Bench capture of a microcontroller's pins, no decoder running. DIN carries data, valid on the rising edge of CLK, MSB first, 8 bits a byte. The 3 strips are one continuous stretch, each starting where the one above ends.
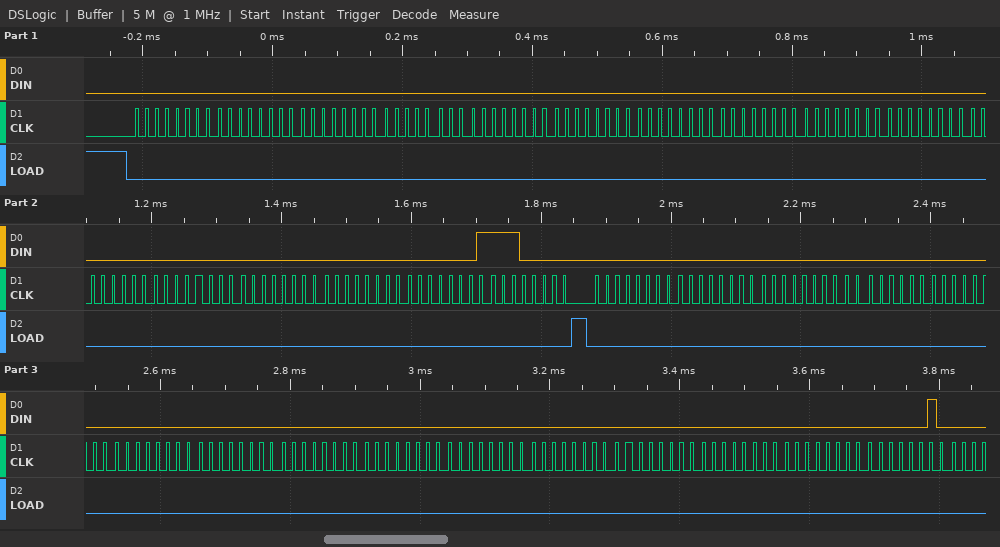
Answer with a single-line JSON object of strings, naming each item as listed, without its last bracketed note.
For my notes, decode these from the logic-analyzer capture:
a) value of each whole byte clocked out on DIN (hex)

{"value of each whole byte clocked out on DIN": "00 00 00 00 00 00 00 00 00 00 00 00 00 00 01 E0 00 00 00 00 00 00 00 00 00 00 00 00 00 00 02"}
